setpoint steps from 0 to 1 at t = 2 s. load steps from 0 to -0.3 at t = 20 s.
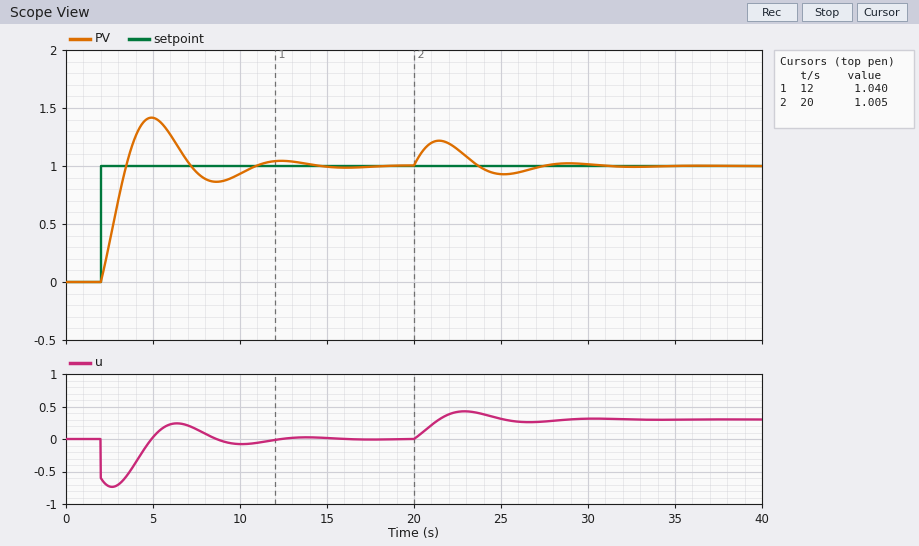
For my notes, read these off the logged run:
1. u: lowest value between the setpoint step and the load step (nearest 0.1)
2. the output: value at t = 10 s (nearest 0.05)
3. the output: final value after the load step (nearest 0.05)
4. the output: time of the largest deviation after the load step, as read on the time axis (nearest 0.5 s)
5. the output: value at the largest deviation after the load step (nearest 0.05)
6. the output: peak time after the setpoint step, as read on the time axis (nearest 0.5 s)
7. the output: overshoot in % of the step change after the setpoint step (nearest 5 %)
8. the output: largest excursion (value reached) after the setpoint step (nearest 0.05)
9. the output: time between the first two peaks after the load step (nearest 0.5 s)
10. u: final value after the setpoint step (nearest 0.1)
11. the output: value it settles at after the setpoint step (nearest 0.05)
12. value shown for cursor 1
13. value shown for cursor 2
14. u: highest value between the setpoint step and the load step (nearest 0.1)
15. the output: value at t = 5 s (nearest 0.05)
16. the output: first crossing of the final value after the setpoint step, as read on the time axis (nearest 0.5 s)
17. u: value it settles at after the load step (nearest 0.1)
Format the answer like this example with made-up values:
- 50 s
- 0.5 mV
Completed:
- -0.7
- 0.95
- 1.00
- 21.5 s
- 1.20
- 5.0 s
- 40 %
- 1.40
- 7.5 s
- 0.0
- 1.00
- 1.040
- 1.005
- 0.2
- 1.40
- 3.5 s
- 0.3
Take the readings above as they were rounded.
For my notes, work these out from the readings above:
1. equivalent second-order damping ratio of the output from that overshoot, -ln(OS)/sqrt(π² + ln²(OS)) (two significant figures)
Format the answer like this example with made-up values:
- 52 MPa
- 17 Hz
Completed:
- 0.28
